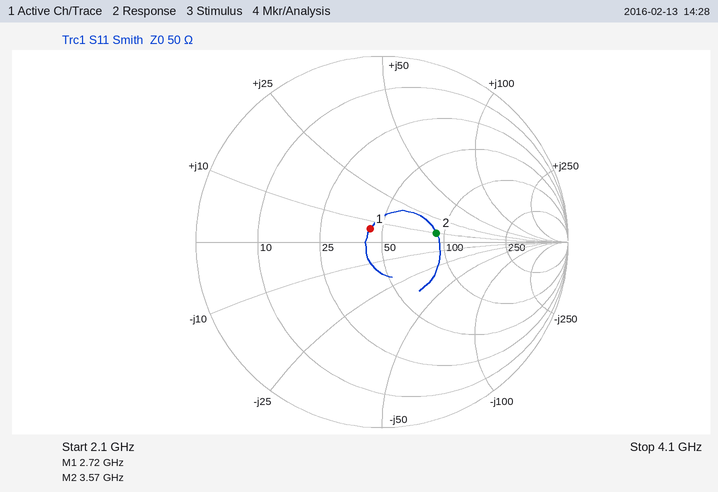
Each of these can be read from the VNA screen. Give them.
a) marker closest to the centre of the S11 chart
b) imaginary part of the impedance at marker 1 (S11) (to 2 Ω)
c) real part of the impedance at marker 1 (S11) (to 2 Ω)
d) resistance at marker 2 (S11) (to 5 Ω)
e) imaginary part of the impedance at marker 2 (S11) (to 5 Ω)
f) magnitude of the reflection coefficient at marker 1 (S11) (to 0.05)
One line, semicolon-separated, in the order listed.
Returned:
marker 1; +6 Ω; 44 Ω; 90 Ω; +10 Ω; 0.10
